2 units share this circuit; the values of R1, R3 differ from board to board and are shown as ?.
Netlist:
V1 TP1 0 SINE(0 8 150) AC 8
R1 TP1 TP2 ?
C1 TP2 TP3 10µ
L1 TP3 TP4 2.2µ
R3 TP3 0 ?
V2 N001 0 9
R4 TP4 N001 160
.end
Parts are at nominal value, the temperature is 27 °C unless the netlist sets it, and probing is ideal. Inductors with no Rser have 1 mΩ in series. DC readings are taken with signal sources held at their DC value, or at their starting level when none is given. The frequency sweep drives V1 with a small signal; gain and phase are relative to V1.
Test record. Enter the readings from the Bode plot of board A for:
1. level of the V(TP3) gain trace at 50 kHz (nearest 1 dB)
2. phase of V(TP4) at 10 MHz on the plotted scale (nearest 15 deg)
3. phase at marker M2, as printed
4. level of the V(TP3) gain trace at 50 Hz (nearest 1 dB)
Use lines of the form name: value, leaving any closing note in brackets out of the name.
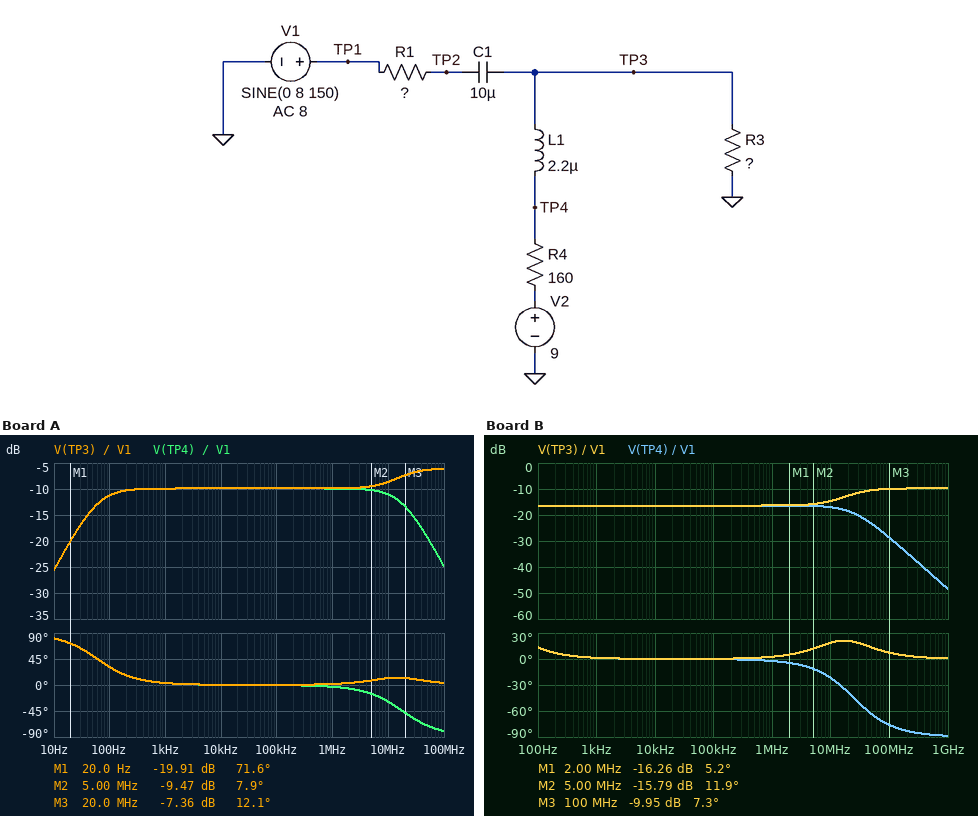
level of the V(TP3) gain trace at 50 kHz: -10 dB
phase of V(TP4) at 10 MHz on the plotted scale: -30 deg
phase at marker M2, as printed: 7.9 deg
level of the V(TP3) gain trace at 50 Hz: -14 dB
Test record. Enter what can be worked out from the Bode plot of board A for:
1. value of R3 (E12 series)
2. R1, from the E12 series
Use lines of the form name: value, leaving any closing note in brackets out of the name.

value of R3: 180 Ω
R1, from the E12 series: 180 Ω
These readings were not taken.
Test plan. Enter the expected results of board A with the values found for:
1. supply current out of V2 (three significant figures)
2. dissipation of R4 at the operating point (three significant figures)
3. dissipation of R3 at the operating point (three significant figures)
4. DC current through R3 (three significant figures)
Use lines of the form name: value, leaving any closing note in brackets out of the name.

supply current out of V2: 26.5 mA
dissipation of R4 at the operating point: 112 mW
dissipation of R3 at the operating point: 126 mW
DC current through R3: 26.5 mA
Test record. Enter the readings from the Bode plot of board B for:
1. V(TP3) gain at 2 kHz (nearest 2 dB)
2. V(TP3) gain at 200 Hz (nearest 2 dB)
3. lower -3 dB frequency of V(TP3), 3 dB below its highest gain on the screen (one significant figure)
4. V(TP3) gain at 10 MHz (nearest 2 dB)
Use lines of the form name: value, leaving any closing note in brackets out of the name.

V(TP3) gain at 2 kHz: -16 dB
V(TP3) gain at 200 Hz: -16 dB
lower -3 dB frequency of V(TP3), 3 dB below its highest gain on the screen: 20 MHz
V(TP3) gain at 10 MHz: -14 dB
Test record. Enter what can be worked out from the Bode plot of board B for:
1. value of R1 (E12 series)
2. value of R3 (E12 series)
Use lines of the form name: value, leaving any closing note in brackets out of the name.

value of R1: 560 Ω
value of R3: 270 Ω
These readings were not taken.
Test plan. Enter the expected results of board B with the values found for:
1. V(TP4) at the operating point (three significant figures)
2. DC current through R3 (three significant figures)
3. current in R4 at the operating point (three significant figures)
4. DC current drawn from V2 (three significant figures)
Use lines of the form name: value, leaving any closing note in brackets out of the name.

V(TP4) at the operating point: 5.65 V
DC current through R3: 20.9 mA
current in R4 at the operating point: 20.9 mA
DC current drawn from V2: 20.9 mA
